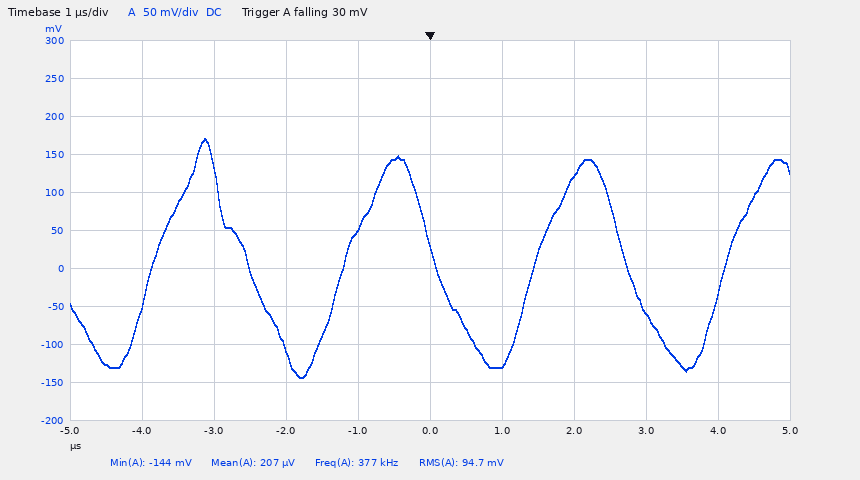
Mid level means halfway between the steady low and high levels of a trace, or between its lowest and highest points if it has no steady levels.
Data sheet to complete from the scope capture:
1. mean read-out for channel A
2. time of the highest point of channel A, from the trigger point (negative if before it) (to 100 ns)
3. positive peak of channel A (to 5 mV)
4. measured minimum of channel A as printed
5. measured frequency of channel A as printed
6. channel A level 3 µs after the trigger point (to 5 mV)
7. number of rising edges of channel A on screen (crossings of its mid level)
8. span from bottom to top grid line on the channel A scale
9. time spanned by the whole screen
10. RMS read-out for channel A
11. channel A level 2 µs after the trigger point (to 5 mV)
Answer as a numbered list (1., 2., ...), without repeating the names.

1. 207 µV
2. -3.1 µs
3. 170 mV
4. -144 mV
5. 377 kHz
6. -60 mV
7. 4
8. 500 mV
9. 10 µs
10. 94.7 mV
11. 120 mV
